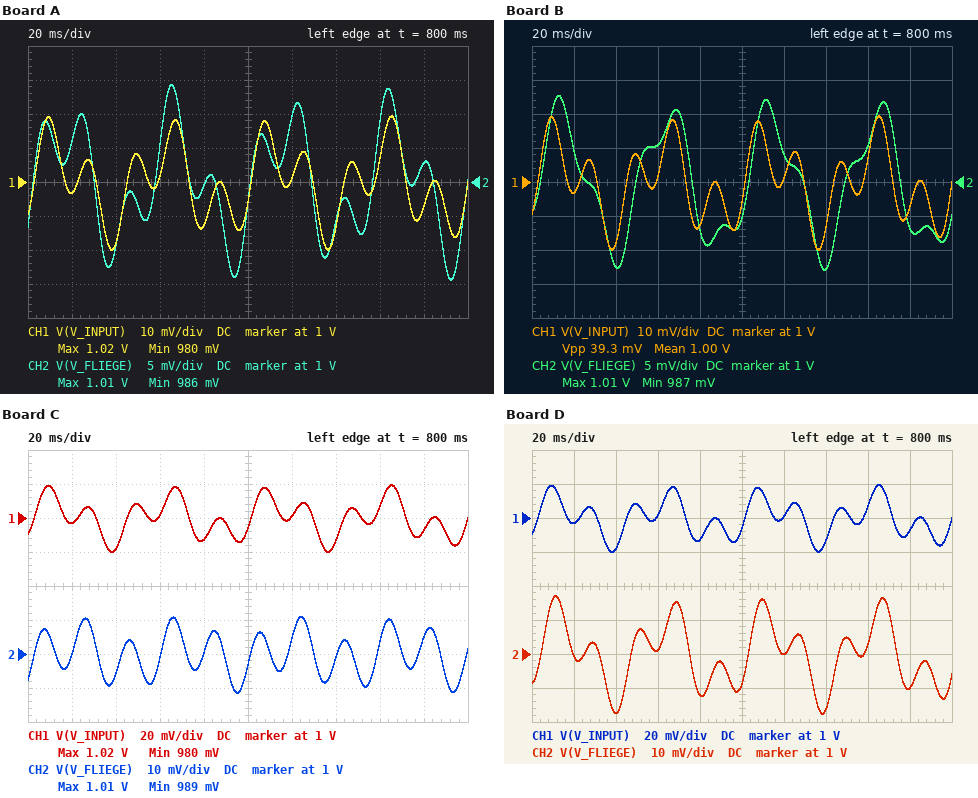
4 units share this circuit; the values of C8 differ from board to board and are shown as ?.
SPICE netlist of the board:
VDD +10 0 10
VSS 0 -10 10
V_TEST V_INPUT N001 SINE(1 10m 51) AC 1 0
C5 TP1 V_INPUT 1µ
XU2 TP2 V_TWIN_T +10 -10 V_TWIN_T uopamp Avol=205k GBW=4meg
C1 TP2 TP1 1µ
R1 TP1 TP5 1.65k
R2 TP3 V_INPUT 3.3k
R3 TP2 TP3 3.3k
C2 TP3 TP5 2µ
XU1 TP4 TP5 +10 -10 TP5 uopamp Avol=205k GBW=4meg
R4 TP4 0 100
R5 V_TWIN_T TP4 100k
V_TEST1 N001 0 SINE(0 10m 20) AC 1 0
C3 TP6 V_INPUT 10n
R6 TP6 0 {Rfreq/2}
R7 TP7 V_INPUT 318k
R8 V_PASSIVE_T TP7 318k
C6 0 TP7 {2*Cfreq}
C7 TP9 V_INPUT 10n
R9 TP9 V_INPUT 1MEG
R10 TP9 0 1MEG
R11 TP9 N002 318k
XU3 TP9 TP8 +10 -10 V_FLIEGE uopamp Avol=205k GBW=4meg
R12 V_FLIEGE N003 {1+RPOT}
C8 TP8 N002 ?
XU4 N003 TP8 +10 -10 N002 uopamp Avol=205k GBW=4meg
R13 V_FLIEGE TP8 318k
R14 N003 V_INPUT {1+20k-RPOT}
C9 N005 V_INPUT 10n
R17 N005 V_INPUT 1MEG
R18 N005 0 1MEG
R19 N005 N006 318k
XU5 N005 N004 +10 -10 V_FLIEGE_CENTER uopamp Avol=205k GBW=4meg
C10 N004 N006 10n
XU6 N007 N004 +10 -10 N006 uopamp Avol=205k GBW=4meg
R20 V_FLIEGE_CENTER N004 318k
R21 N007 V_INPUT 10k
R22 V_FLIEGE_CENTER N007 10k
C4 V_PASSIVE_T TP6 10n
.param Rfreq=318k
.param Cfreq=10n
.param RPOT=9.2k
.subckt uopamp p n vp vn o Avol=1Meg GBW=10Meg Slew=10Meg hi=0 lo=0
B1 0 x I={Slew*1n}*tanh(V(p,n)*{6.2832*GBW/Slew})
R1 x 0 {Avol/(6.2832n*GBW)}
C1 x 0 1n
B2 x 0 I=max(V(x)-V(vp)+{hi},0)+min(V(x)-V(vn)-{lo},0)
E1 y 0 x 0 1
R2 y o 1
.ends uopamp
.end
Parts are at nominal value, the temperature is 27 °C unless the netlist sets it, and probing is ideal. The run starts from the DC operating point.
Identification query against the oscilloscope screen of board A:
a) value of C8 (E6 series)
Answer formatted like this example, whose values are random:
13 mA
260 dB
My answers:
15 nF
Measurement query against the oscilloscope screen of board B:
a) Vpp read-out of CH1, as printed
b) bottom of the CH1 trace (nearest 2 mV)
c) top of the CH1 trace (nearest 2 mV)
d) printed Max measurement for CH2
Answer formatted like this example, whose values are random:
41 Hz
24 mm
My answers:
39.3 mV
980 mV
1.020 V
1.01 V
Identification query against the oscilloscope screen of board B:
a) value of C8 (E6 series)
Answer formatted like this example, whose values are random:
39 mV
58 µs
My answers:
6.8 nF
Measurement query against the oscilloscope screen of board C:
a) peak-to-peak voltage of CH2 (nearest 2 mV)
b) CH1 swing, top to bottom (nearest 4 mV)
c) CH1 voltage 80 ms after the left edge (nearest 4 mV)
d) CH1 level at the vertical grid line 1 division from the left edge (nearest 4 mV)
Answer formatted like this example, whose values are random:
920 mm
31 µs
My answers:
22 mV
40 mV
988 mV
996 mV
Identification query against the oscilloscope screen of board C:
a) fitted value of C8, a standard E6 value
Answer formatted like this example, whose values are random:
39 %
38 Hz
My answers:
33 nF
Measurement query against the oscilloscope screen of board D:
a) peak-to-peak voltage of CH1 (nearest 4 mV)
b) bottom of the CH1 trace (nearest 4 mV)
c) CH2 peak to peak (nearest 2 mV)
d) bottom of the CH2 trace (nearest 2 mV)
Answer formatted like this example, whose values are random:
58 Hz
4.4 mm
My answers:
40 mV
980 mV
34 mV
982 mV
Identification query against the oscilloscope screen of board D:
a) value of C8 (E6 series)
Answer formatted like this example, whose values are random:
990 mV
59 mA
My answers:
4.7 nF
